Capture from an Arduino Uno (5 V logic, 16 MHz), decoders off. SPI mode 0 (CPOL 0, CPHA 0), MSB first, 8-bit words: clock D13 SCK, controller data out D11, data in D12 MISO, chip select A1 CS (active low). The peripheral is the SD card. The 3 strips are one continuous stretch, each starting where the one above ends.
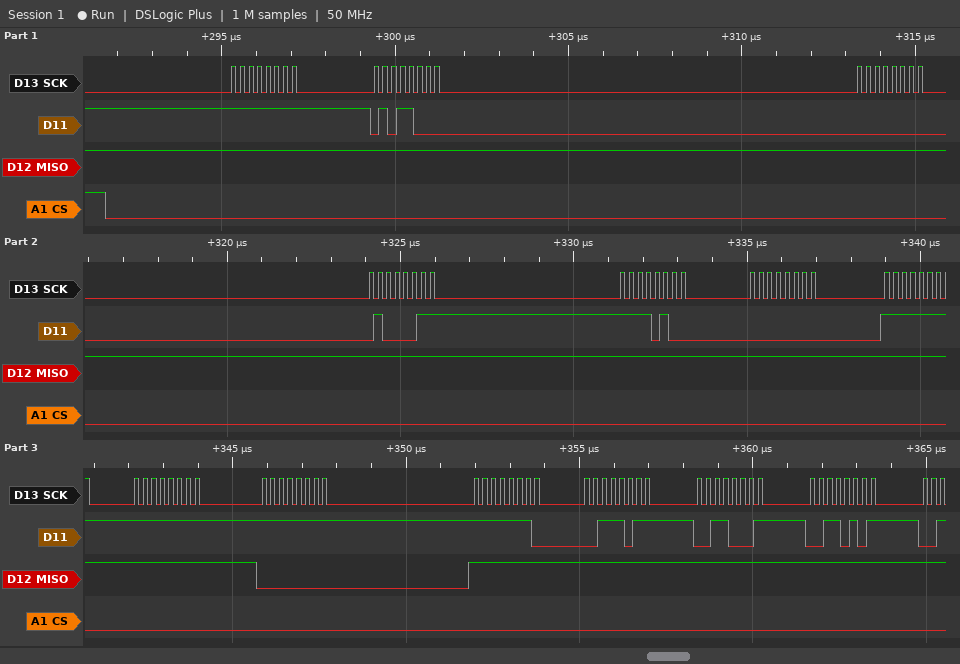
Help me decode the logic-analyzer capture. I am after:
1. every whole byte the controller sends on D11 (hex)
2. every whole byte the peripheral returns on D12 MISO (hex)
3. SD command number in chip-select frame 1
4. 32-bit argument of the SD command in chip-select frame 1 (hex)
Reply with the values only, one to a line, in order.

0xFF 0x58 0x00 0x43 0xF4 0x00 0xFF 0xFF 0xFF 0xFE 0x3B 0x31 0x35
0xFF 0xFF 0xFF 0xFF 0xFF 0xFF 0xFF 0xFF 0x00 0xFF 0xFF 0xFF 0xFF
CMD24
0x0043F400
